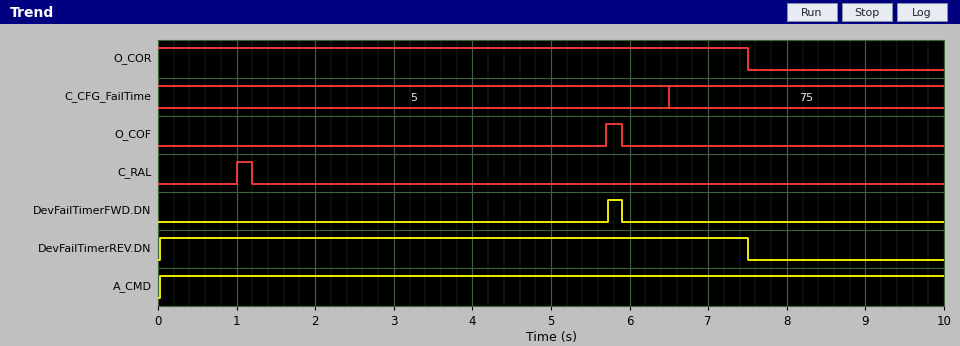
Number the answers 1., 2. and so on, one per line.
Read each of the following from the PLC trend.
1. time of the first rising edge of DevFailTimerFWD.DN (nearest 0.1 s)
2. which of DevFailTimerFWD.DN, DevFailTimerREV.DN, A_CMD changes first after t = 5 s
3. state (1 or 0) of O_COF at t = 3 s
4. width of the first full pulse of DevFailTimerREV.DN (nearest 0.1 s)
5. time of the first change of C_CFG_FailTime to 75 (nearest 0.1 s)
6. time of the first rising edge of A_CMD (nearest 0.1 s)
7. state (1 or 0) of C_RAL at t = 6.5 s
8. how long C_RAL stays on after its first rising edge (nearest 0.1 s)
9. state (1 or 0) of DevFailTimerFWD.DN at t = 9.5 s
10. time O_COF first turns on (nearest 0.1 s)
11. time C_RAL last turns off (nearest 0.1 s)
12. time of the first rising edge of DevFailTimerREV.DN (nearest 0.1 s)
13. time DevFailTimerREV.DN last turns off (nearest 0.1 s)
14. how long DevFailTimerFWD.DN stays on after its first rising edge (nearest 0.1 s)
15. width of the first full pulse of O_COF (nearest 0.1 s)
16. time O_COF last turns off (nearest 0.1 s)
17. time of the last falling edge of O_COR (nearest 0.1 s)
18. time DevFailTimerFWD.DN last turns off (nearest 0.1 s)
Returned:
1. 5.7 s
2. DevFailTimerFWD.DN
3. 0
4. 7.5 s
5. 6.5 s
6. 0.0 s
7. 0
8. 0.2 s
9. 0
10. 5.7 s
11. 1.2 s
12. 0.0 s
13. 7.5 s
14. 0.2 s
15. 0.2 s
16. 5.9 s
17. 7.5 s
18. 5.9 s
